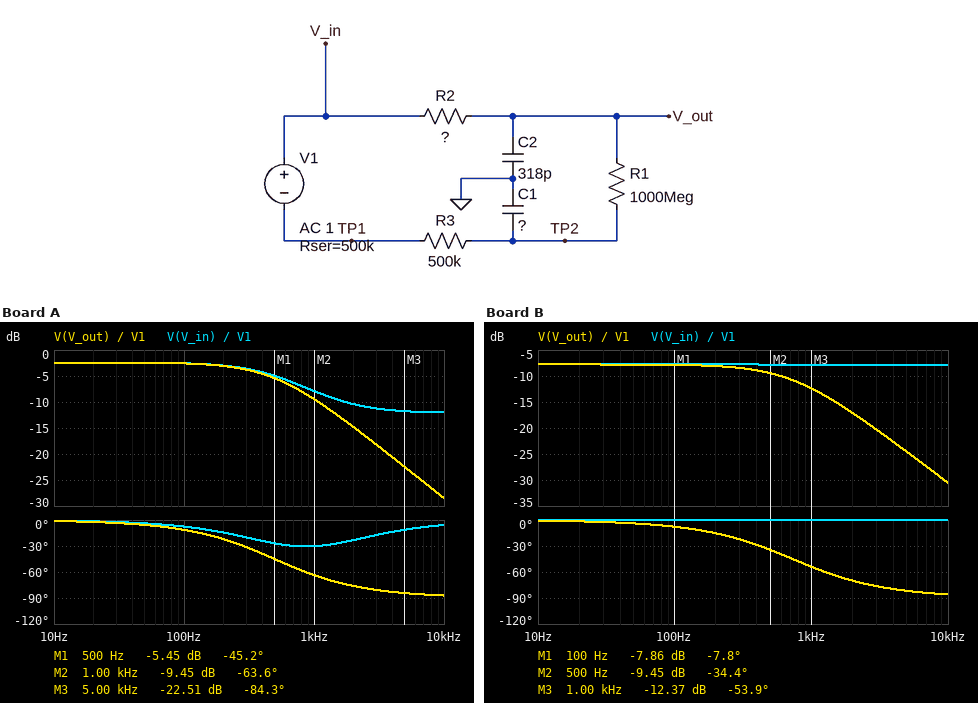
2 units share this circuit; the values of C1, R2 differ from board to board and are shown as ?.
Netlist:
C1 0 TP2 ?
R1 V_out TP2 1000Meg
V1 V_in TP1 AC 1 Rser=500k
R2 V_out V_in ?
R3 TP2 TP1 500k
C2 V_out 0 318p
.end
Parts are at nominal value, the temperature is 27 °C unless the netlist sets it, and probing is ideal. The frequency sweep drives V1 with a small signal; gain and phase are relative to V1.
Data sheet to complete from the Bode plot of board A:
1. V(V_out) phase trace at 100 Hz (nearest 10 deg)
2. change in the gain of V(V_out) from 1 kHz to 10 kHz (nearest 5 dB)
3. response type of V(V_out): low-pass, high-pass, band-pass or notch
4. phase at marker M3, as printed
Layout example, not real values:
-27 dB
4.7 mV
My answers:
-10 deg
-20 dB
low-pass
-84.3 deg
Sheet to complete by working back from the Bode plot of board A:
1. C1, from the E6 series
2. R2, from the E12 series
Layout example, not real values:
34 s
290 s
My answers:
1 nF
330 kΩ
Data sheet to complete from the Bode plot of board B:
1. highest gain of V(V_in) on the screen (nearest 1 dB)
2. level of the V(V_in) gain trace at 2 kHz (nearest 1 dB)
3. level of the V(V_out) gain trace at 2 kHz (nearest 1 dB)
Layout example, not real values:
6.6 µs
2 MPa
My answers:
-8 dB
-8 dB
-17 dB
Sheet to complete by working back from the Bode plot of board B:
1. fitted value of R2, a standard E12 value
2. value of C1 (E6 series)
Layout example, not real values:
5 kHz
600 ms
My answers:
680 kΩ
220 pF
